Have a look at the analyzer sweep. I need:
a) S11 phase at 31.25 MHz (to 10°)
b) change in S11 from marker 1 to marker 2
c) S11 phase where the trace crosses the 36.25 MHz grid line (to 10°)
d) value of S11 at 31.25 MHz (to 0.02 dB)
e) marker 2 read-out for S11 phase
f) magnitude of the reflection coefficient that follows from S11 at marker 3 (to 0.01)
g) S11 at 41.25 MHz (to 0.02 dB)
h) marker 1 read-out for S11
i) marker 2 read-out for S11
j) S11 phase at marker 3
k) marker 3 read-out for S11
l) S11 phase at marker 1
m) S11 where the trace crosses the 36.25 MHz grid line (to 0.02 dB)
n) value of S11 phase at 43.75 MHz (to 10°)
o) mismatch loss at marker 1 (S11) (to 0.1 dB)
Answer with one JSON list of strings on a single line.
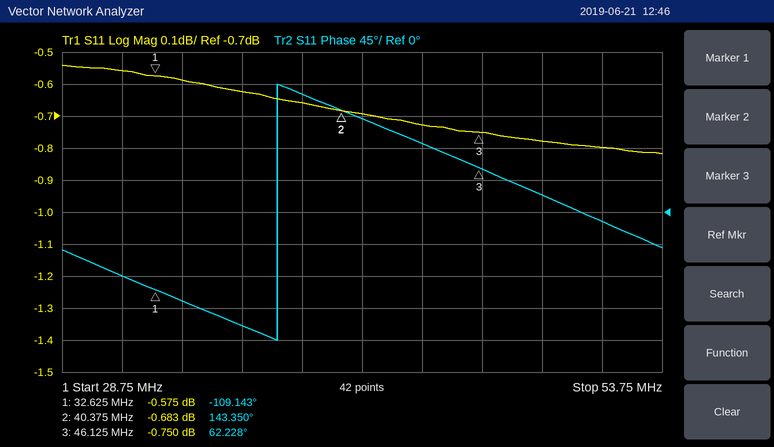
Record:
["-90°", "-0.108 dB", "-160°", "-0.56 dB", "143.350°", "0.92", "-0.70 dB", "-0.575 dB", "-0.683 dB", "62.228°", "-0.750 dB", "-109.143°", "-0.62 dB", "100°", "9.1 dB"]
